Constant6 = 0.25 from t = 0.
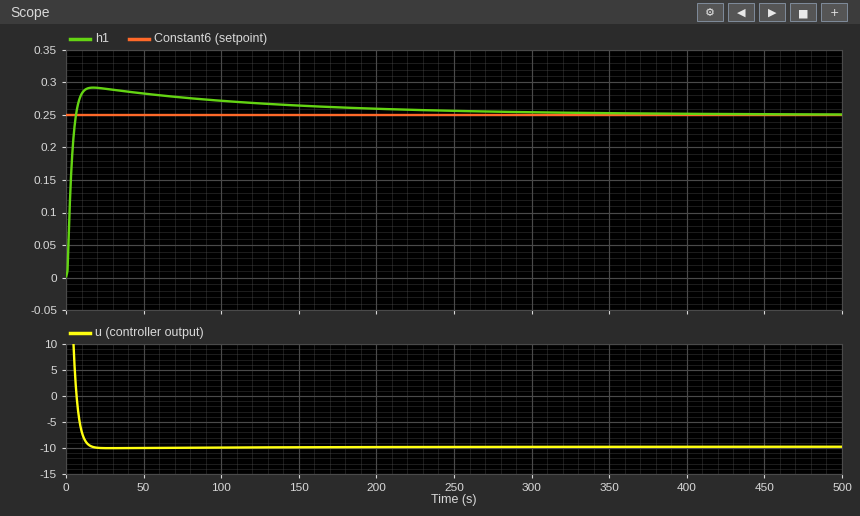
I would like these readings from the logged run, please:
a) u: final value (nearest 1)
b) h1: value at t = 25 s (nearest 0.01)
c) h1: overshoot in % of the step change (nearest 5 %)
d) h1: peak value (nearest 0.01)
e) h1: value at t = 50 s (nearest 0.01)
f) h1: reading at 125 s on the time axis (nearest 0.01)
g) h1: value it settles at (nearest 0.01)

-10
0.29
15 %
0.29
0.28
0.27
0.25
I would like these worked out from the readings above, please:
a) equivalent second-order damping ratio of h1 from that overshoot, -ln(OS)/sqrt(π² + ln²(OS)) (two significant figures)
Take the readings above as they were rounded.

0.52
